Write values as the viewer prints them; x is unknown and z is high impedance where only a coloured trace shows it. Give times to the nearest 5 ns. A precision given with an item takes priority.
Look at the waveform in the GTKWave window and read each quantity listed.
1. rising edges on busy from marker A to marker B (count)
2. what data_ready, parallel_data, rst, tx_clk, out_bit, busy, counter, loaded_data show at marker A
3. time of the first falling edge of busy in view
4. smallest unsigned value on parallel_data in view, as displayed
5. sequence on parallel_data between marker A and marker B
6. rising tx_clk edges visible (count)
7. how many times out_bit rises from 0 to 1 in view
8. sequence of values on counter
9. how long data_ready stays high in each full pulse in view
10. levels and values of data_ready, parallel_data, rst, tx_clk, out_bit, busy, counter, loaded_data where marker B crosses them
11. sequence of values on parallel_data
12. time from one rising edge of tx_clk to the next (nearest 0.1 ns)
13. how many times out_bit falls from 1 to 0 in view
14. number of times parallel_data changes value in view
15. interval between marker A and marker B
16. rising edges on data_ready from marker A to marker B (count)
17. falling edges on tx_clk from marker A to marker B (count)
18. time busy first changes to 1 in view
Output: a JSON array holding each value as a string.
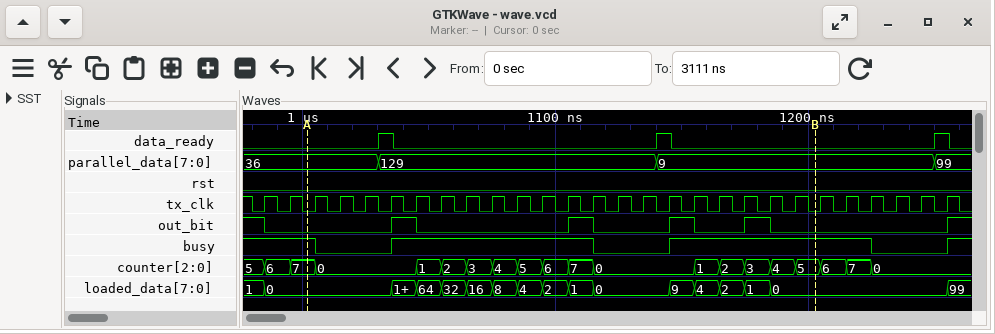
["2", "data_ready=0, parallel_data=36, rst=0, tx_clk=0, out_bit=0, busy=1, counter=7, loaded_data=0", "1005 ns", "9", "36, 129, 9", "28", "5", "5, 6, 7, 0, 1, 2, 3, 4, 5, 6, 7, 0, 1, 2, 3, 4, 5, 6, 7, 0", "5 ns, 5 ns, 5 ns", "data_ready=0, parallel_data=9, rst=0, tx_clk=0, out_bit=0, busy=1, counter=5, loaded_data=0", "36, 129, 9, 99", "10 ns", "5", "3", "200 ns", "2", "20", "1035 ns"]
